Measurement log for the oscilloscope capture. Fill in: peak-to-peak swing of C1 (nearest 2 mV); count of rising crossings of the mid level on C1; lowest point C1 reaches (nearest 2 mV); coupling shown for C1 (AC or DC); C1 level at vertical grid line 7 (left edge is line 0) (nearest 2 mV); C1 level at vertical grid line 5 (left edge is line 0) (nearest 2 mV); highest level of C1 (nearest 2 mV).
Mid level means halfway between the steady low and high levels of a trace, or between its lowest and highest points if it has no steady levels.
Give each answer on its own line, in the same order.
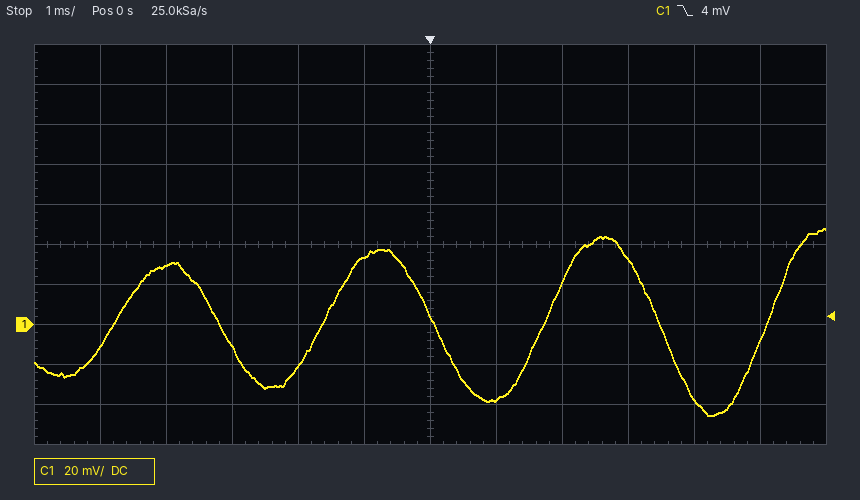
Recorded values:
94 mV
4
-46 mV
DC
-38 mV
34 mV
48 mV
